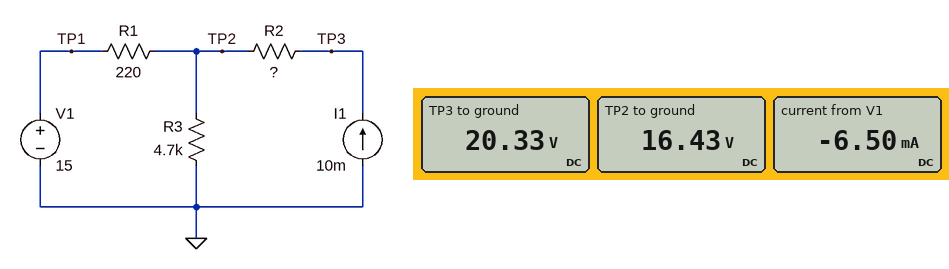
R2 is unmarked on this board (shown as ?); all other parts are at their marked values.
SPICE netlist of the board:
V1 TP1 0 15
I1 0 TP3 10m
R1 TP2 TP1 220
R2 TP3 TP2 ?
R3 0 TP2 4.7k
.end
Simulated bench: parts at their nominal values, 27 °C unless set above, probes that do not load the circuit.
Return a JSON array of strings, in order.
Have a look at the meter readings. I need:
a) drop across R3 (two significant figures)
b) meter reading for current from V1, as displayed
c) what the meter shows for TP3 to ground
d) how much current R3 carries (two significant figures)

["16 V", "-6.50 mA", "20.33 V", "3.5 mA"]
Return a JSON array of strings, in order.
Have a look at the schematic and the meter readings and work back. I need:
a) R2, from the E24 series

["390 Ω"]
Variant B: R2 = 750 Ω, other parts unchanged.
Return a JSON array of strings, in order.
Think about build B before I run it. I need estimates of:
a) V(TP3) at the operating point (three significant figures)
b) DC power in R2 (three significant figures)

["23.9 V", "75.0 mW"]
